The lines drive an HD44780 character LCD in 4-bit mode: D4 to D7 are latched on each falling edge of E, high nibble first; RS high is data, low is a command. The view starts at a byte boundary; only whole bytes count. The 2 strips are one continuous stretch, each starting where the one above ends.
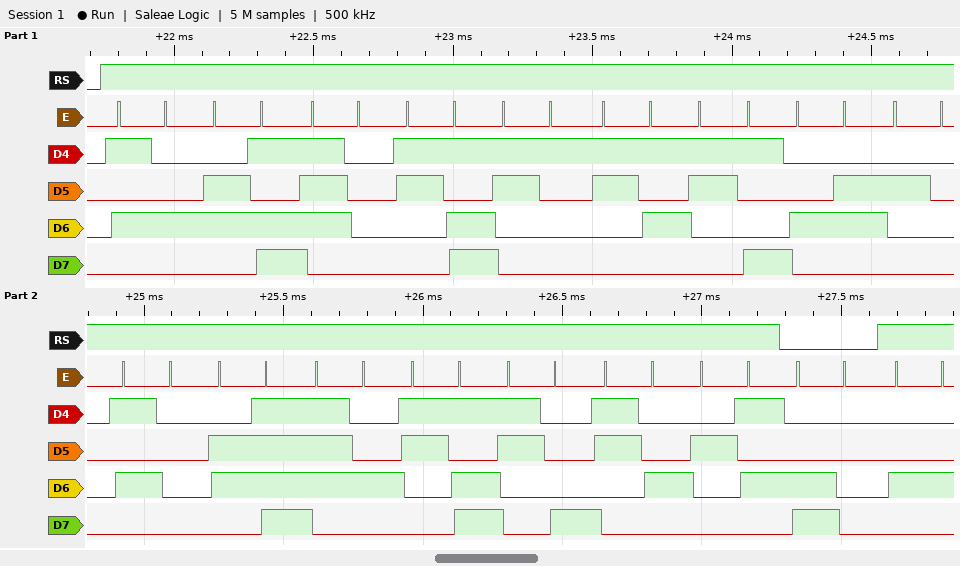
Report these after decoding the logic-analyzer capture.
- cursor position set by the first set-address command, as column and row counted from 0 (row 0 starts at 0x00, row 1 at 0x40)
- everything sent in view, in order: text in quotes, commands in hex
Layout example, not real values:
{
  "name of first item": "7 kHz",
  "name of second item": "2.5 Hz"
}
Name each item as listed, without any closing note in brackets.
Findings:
{
  "cursor position set by the first set-address command, as column and row counted from 0": "column 0, row 1",
  "everything sent in view, in order: text in quotes, commands in hex": "\"Tmp=159F Pot=84%\" 0xC0 \"D\""
}
